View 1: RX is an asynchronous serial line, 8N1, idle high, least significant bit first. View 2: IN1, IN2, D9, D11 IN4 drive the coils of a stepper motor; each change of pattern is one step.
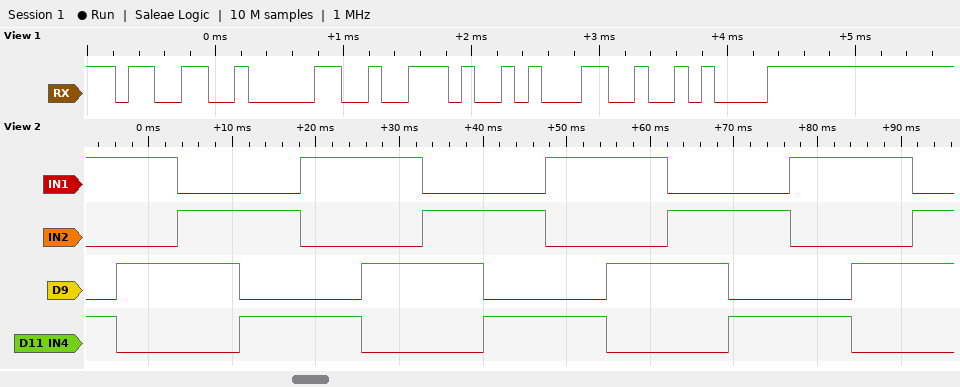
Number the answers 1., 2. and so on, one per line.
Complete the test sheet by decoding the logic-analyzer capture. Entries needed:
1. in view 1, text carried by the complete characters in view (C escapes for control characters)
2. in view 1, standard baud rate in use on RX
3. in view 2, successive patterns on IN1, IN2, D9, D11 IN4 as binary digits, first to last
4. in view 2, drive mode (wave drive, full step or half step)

1. "30.1\n"
2. 9600 baud
3. 1001 1010 0110 0101 1001 1010 0110 0101 1001 1010 0110 0101 1001 1010 0110
4. full step
